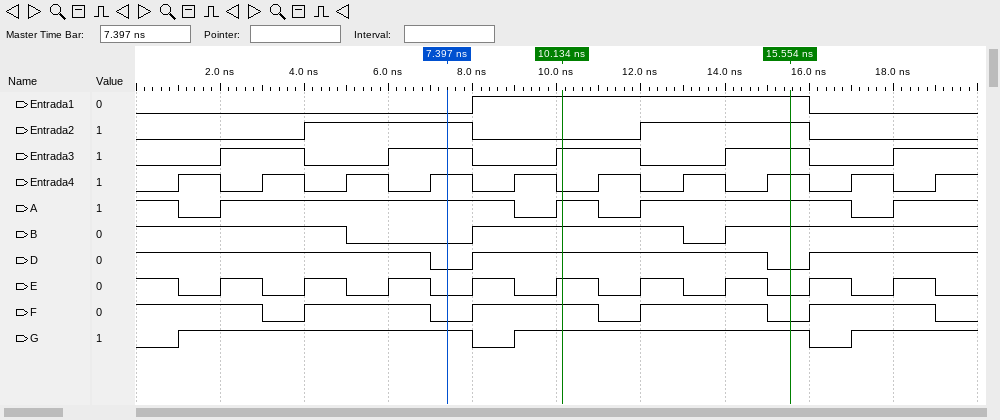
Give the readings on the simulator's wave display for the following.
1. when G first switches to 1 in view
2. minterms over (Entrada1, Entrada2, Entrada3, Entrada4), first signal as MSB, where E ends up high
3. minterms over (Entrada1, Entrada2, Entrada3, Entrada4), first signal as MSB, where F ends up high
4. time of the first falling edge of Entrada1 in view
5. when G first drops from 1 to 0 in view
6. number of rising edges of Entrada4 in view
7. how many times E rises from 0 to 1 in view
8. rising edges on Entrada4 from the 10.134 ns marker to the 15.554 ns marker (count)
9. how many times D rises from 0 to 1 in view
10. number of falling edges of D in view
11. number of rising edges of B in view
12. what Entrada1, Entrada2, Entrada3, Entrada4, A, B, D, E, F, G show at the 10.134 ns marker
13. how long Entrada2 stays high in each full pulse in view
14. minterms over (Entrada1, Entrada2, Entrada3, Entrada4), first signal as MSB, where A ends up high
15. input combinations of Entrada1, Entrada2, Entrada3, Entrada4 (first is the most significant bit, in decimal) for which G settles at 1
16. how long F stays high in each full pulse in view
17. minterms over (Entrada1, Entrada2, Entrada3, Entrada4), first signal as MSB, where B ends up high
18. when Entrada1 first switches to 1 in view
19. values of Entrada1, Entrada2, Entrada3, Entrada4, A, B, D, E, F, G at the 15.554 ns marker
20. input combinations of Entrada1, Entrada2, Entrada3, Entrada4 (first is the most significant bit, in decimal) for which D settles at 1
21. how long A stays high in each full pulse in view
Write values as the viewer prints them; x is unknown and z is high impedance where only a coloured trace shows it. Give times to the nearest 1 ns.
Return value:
1 ns
0, 2, 4, 6, 8, 10, 12, 14
0, 1, 2, 4, 5, 6, 8, 9, 10, 12, 13, 14
16 ns
8 ns
10
9
3
2
2
2
Entrada1=1, Entrada2=0, Entrada3=1, Entrada4=0, A=1, B=1, D=1, E=1, F=1, G=1
4 ns, 4 ns
0, 2, 3, 4, 5, 6, 7, 8, 10, 12, 13, 14, 15
1, 2, 3, 4, 5, 6, 7, 9, 10, 11, 12, 13, 14, 15
3 ns, 3 ns, 3 ns, 3 ns
0, 1, 2, 3, 4, 8, 9, 10, 11, 12, 14, 15
8 ns
Entrada1=1, Entrada2=1, Entrada3=1, Entrada4=1, A=1, B=1, D=0, E=0, F=0, G=1
0, 1, 2, 3, 4, 5, 6, 8, 9, 10, 11, 12, 13, 14
7 ns, 1 ns, 5 ns
